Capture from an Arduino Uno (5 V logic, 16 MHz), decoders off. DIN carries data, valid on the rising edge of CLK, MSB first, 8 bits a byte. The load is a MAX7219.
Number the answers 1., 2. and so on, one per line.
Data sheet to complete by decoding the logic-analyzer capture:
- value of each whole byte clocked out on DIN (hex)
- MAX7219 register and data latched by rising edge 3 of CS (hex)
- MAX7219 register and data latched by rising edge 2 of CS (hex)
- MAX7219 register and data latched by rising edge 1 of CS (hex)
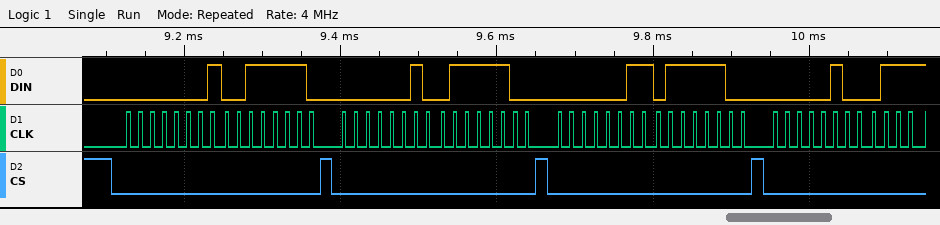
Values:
1. 01 3E 02 7C 03 7C 04
2. register 0x3, data 0x7C
3. register 0x2, data 0x7C
4. register 0x1, data 0x3E
